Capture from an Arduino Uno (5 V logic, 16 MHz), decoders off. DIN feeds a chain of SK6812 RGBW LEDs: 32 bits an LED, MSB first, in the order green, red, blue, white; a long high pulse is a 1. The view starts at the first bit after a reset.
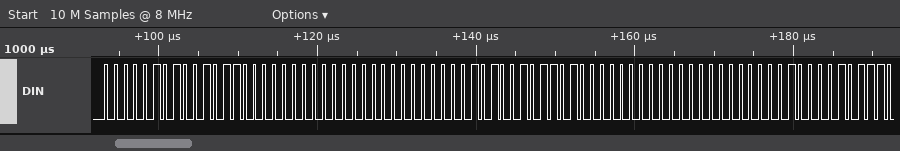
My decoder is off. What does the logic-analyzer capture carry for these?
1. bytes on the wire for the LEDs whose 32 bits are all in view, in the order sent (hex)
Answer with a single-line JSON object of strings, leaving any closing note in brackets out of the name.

{"bytes on the wire for the LEDs whose 32 bits are all in view, in the order sent": "05 2C 00 00 05 2D 00 00"}
